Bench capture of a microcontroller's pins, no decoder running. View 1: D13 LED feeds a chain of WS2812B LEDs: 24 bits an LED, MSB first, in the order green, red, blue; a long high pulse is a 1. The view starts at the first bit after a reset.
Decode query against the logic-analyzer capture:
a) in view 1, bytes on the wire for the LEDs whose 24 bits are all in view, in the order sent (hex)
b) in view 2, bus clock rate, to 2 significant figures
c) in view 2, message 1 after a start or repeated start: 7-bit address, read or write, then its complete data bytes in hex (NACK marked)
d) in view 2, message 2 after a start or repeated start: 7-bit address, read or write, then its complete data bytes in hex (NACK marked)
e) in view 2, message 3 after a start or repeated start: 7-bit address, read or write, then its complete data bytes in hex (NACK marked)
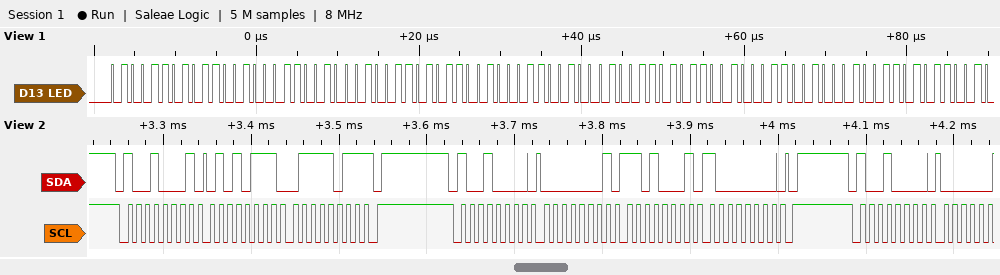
4D 64 64 4D 64 64 4D 64 64
100 kHz
0x48 read: 57 7B NACK
0x48 write: 01 D1 80
0x48 write
